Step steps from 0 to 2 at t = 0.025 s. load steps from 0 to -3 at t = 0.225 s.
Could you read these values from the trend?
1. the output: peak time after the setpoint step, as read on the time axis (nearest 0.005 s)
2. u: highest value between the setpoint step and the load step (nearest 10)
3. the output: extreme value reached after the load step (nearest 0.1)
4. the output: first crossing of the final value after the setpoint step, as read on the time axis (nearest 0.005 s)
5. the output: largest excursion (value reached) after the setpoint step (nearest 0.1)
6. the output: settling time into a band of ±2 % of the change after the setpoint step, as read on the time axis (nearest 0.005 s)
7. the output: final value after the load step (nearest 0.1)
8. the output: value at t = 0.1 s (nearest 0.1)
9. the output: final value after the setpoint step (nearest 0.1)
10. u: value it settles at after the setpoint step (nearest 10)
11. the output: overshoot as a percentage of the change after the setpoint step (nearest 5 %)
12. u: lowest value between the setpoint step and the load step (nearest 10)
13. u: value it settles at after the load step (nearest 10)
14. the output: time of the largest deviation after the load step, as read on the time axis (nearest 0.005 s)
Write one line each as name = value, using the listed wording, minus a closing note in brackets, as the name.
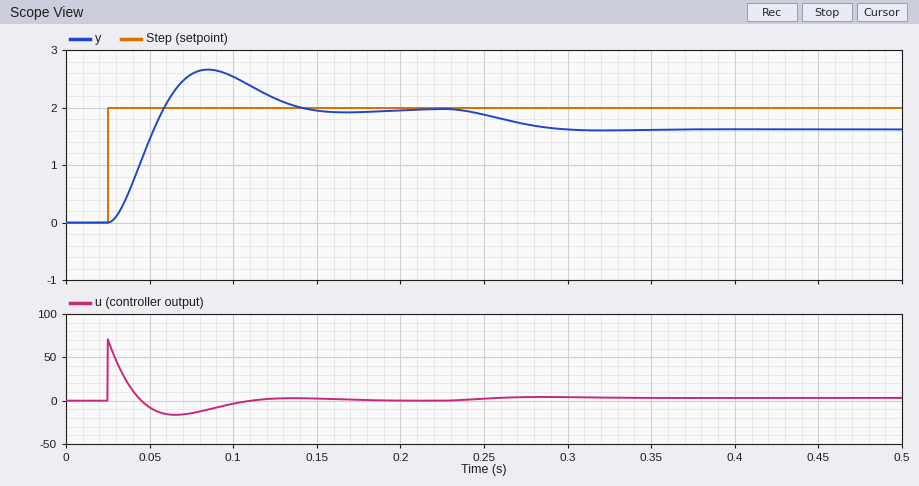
the output: peak time after the setpoint step, as read on the time axis = 0.085 s
u: highest value between the setpoint step and the load step = 70
the output: extreme value reached after the load step = 1.6
the output: first crossing of the final value after the setpoint step, as read on the time axis = 0.060 s
the output: largest excursion (value reached) after the setpoint step = 2.7
the output: settling time into a band of ±2 % of the change after the setpoint step, as read on the time axis = 0.185 s
the output: final value after the load step = 1.6
the output: value at t = 0.1 s = 2.5
the output: final value after the setpoint step = 2.0
u: value it settles at after the setpoint step = 0
the output: overshoot as a percentage of the change after the setpoint step = 35 %
u: lowest value between the setpoint step and the load step = -20
u: value it settles at after the load step = 0
the output: time of the largest deviation after the load step, as read on the time axis = 0.320 s
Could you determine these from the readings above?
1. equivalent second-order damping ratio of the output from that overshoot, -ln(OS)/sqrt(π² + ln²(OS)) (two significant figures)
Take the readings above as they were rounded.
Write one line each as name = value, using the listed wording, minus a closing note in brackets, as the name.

equivalent second-order damping ratio of the output from that overshoot, -ln(OS)/sqrt(π² + ln²(OS)) = 0.32
